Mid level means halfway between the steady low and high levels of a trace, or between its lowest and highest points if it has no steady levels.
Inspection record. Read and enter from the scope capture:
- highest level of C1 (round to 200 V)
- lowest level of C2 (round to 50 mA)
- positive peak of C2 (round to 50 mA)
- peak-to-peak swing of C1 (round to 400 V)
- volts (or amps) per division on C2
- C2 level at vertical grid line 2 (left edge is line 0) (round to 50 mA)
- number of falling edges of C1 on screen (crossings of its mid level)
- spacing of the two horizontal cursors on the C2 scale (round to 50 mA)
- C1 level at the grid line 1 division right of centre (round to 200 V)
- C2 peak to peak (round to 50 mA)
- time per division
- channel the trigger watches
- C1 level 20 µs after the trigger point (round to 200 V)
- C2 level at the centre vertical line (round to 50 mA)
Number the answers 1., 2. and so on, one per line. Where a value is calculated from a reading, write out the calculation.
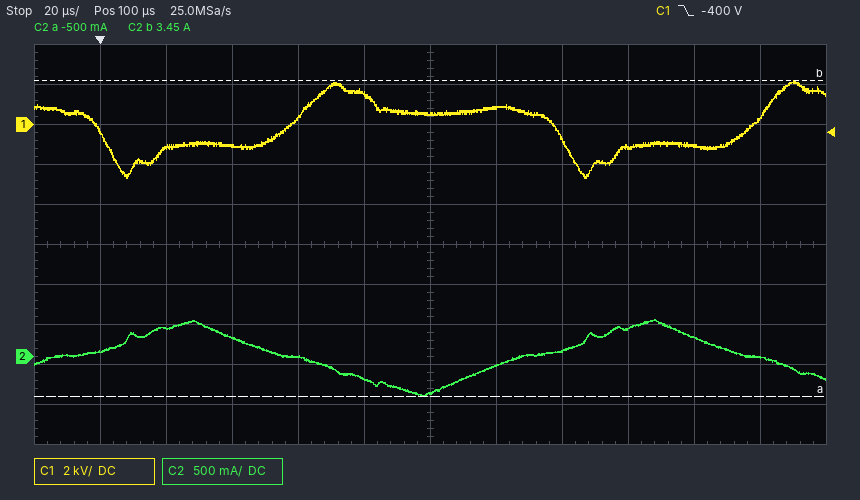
1. 2.2 kV
2. -500 mA
3. 450 mA
4. 4.8 kV
5. 500 mA
6. 350 mA
7. 2
8. 3.95 A
9. 800 V
10. 450 mA − (-500 mA) = 950 mA
11. 20 µs
12. C1
13. -1.2 kV
14. -450 mA
